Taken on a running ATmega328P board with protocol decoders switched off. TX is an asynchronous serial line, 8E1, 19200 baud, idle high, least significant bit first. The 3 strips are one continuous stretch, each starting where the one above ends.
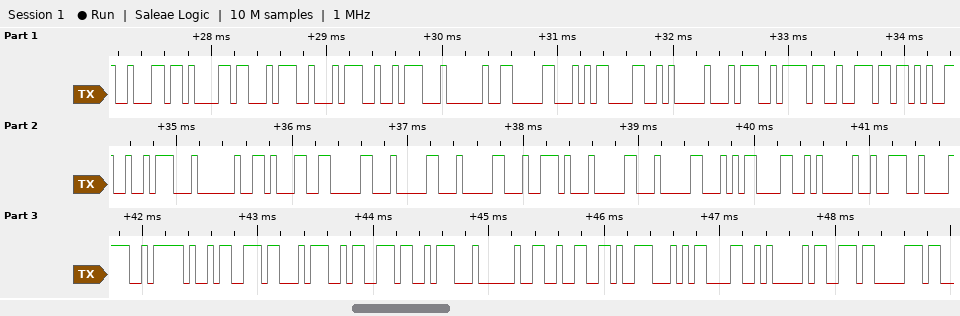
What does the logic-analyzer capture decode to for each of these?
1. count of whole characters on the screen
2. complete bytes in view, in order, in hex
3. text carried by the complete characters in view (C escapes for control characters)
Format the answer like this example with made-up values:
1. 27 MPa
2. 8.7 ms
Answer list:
1. 38
2. 62 61 74 74 3A 20 30 0D 0A 74 6F 6E 65 3A 20 31 30 30 30 2E 30 30 0D 0A 72 78 5F 73 74 73 3A 20 32 39 0D 0A 73 70
3. "batt: 0\r\ntone: 1000.00\r\nrx_sts: 29\r\nsp"
